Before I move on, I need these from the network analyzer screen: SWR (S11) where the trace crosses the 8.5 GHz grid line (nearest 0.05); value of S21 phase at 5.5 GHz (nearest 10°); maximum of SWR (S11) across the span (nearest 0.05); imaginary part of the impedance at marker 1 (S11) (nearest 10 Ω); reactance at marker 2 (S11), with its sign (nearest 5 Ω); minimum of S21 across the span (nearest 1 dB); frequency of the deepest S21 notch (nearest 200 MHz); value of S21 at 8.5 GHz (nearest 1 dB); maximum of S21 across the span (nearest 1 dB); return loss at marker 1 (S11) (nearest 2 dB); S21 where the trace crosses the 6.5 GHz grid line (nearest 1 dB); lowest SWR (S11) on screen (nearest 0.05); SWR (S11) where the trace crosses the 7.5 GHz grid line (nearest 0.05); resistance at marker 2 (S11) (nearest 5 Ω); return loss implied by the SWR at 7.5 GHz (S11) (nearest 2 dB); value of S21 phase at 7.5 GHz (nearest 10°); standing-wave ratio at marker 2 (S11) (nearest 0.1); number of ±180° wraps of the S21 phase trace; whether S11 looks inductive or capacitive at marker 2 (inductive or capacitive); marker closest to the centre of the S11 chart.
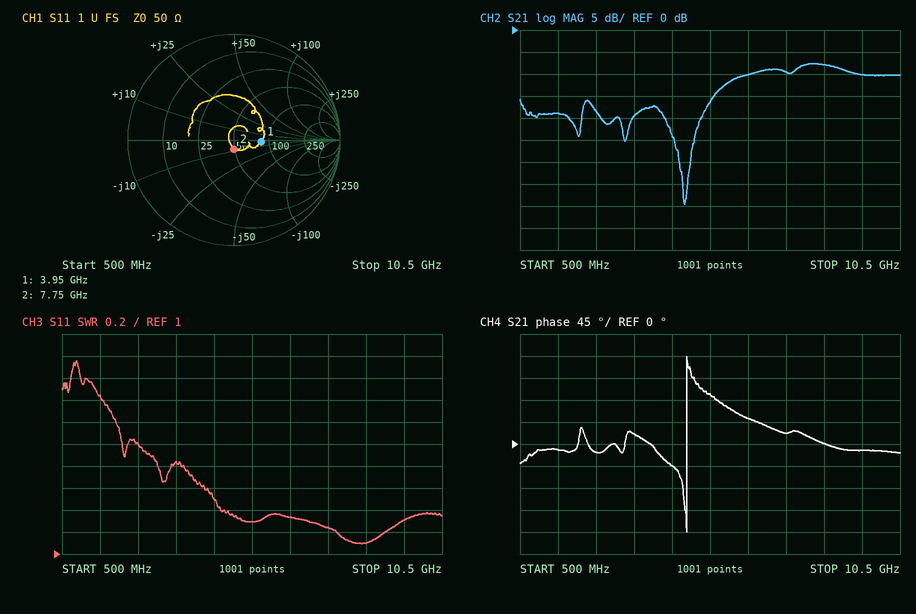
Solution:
1.10
100°
2.75
0 Ω
-10 Ω
-40 dB
4.8 GHz
-8 dB
-8 dB
12 dB
-10 dB
1.10
1.25
50 Ω
20 dB
20°
1.2
1
capacitive
marker 2
